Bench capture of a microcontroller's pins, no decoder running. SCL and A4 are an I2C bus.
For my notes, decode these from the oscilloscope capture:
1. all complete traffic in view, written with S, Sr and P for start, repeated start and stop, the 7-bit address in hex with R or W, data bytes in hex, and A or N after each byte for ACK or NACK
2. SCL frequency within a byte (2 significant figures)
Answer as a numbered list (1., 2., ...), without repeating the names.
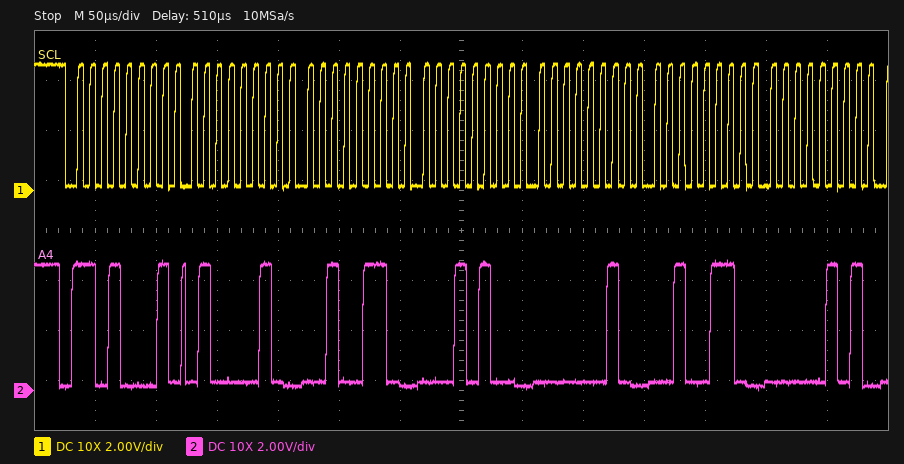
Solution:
1. S 68R A 42 A 26 A 14 A 02 A 26 A 05 A
2. 100 kHz
